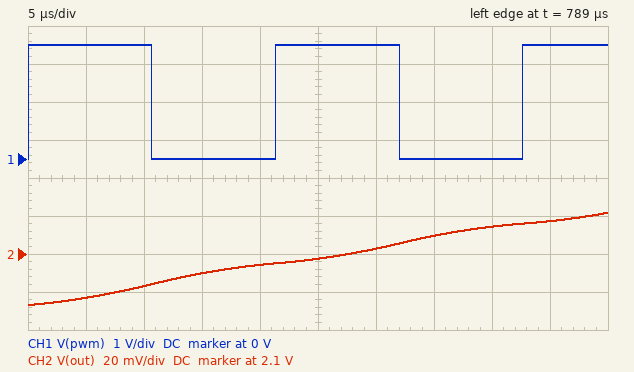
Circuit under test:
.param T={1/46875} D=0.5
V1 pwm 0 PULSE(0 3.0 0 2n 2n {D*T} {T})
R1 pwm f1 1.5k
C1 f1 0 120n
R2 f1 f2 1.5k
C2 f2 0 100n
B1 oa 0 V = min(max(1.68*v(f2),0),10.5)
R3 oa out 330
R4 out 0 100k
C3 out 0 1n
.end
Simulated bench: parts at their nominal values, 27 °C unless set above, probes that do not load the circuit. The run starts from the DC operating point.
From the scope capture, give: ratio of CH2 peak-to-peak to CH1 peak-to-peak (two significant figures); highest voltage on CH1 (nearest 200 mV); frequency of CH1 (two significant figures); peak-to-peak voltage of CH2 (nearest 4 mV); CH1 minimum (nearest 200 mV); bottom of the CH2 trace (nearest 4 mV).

0.016
3.0 V
47 kHz
48 mV
0 V
2.072 V
